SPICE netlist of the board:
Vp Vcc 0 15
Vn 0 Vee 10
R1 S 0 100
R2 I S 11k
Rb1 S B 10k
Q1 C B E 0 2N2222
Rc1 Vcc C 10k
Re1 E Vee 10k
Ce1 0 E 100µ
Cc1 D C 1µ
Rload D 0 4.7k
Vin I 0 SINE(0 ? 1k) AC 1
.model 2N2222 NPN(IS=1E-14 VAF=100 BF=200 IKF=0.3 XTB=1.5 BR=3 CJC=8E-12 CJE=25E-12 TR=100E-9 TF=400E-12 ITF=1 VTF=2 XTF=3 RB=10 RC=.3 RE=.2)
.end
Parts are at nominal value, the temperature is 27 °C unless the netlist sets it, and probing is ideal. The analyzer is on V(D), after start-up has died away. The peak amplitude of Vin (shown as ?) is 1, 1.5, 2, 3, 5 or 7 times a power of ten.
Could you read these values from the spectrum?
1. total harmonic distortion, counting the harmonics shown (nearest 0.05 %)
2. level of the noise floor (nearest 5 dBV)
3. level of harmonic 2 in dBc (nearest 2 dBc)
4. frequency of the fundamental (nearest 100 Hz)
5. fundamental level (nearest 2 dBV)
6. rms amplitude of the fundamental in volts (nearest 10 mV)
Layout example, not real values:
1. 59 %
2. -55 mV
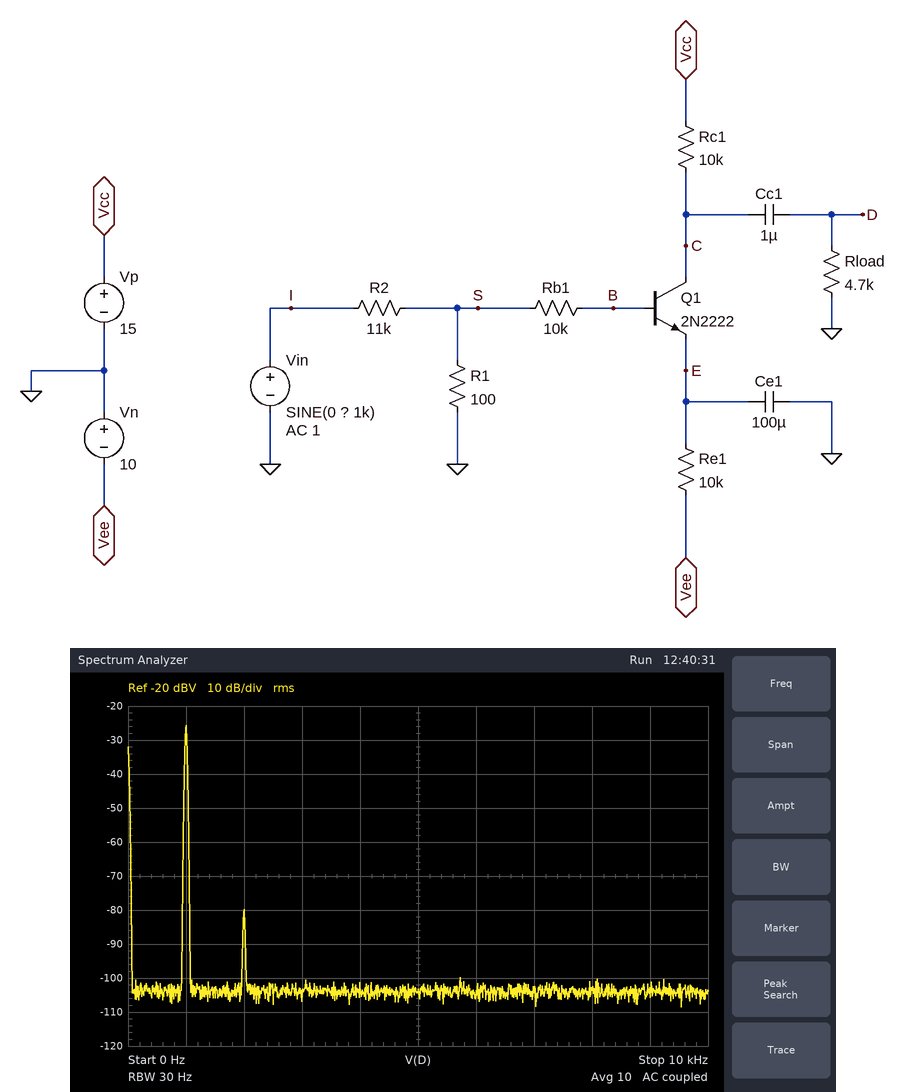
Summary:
1. 0.20 %
2. -105 dBV
3. -54 dBc
4. 1.0 kHz
5. -26 dBV
6. 50 mV
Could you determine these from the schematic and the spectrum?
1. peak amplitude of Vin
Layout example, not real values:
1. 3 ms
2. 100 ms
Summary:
1. 200 mV
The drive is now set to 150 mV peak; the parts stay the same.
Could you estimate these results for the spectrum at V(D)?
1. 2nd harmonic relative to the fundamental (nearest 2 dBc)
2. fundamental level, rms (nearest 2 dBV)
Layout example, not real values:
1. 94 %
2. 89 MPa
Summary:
1. -56 dBc
2. -28 dBV
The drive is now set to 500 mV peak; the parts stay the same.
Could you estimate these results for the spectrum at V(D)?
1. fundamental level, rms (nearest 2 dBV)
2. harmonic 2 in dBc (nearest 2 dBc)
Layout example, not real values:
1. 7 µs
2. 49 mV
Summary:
1. -18 dBV
2. -46 dBc
